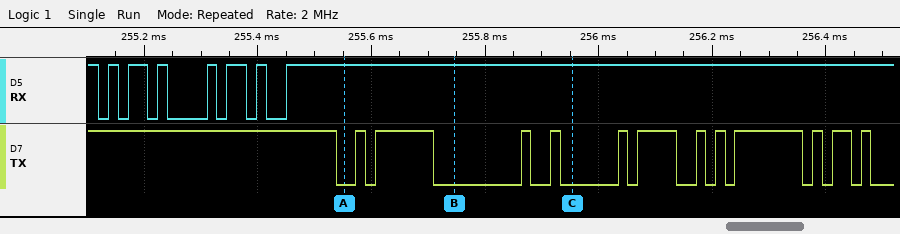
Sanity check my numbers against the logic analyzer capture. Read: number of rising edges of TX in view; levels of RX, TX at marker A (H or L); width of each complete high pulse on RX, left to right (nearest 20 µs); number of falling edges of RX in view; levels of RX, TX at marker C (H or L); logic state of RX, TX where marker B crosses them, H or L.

12
RX=H, TX=L
20 µs, 40 µs, 20 µs, 20 µs, 40 µs, 20 µs
7
RX=H, TX=L
RX=H, TX=L
